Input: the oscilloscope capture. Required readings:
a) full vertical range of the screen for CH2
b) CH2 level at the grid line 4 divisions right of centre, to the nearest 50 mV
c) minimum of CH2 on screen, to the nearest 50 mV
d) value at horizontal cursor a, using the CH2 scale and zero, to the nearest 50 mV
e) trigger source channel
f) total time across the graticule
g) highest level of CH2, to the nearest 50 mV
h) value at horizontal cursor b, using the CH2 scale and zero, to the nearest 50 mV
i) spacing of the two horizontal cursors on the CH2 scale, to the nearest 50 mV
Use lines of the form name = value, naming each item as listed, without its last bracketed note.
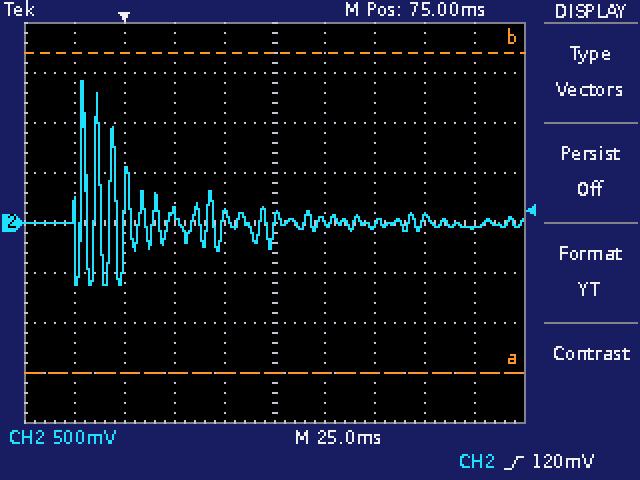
full vertical range of the screen for CH2 = 4 V
CH2 level at the grid line 4 divisions right of centre, to the nearest 50 mV = -50 mV
minimum of CH2 on screen, to the nearest 50 mV = -600 mV
value at horizontal cursor a, using the CH2 scale and zero, to the nearest 50 mV = -1.50 V
trigger source channel = CH2
total time across the graticule = 250 ms
highest level of CH2, to the nearest 50 mV = 1.40 V
value at horizontal cursor b, using the CH2 scale and zero, to the nearest 50 mV = 1.70 V
spacing of the two horizontal cursors on the CH2 scale, to the nearest 50 mV = 3.20 V
